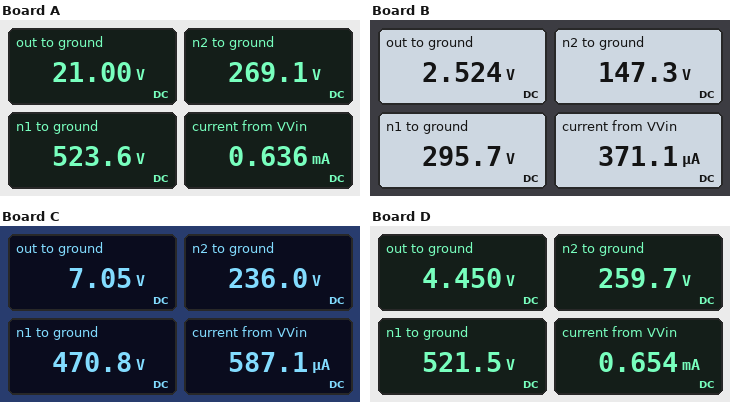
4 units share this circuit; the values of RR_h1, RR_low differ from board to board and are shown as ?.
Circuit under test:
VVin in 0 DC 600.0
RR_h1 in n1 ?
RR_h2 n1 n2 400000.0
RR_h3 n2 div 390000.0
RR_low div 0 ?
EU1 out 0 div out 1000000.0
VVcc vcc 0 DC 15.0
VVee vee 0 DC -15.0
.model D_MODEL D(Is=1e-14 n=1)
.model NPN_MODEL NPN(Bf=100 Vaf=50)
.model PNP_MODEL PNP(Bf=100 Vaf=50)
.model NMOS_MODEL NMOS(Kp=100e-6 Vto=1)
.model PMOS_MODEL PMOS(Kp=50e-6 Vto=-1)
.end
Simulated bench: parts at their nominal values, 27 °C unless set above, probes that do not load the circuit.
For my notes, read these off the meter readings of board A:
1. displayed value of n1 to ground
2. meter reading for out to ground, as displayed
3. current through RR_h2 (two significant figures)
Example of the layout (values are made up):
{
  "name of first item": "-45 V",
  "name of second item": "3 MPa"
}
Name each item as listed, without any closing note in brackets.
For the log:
{
  "displayed value of n1 to ground": "523.6 V",
  "meter reading for out to ground, as displayed": "21.00 V",
  "current through RR_h2": "640 µA"
}
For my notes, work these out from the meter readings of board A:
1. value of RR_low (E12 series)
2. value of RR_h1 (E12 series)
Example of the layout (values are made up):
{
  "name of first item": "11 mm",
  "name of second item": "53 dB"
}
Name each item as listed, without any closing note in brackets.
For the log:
{
  "value of RR_low": "33 kΩ",
  "value of RR_h1": "120 kΩ"
}
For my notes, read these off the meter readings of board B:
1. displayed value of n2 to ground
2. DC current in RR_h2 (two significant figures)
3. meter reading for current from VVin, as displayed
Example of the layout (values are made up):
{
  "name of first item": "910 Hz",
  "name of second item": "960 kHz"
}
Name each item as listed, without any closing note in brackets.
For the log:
{
  "displayed value of n2 to ground": "147.3 V",
  "DC current in RR_h2": "370 µA",
  "meter reading for current from VVin, as displayed": "371.1 µA"
}
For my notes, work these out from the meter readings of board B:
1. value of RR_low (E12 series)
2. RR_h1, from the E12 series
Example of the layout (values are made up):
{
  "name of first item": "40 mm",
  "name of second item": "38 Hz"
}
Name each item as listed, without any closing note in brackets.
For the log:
{
  "value of RR_low": "6.8 kΩ",
  "RR_h1, from the E12 series": "820 kΩ"
}
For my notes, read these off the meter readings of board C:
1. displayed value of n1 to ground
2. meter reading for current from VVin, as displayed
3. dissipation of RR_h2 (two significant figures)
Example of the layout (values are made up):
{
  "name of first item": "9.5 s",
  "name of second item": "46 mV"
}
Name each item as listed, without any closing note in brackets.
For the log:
{
  "displayed value of n1 to ground": "470.8 V",
  "meter reading for current from VVin, as displayed": "587.1 µA",
  "dissipation of RR_h2": "140 mW"
}
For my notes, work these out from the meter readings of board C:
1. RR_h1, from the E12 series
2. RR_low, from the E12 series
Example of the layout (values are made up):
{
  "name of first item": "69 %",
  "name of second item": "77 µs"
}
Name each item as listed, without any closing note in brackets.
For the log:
{
  "RR_h1, from the E12 series": "220 kΩ",
  "RR_low, from the E12 series": "12 kΩ"
}
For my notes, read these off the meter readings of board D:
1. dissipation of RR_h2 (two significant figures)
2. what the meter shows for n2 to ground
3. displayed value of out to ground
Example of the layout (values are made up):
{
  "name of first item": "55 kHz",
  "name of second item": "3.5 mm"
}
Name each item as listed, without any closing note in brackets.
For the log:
{
  "dissipation of RR_h2": "170 mW",
  "what the meter shows for n2 to ground": "259.7 V",
  "displayed value of out to ground": "4.450 V"
}
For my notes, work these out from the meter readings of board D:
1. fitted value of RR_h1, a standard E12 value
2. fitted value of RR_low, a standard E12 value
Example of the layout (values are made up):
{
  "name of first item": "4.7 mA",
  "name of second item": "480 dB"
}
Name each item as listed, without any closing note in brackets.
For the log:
{
  "fitted value of RR_h1, a standard E12 value": "120 kΩ",
  "fitted value of RR_low, a standard E12 value": "6.8 kΩ"
}
